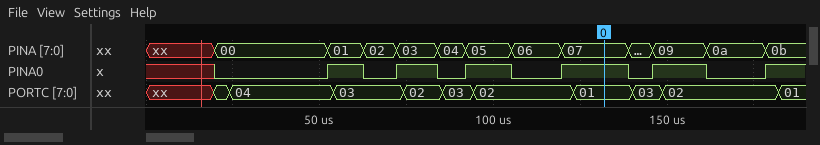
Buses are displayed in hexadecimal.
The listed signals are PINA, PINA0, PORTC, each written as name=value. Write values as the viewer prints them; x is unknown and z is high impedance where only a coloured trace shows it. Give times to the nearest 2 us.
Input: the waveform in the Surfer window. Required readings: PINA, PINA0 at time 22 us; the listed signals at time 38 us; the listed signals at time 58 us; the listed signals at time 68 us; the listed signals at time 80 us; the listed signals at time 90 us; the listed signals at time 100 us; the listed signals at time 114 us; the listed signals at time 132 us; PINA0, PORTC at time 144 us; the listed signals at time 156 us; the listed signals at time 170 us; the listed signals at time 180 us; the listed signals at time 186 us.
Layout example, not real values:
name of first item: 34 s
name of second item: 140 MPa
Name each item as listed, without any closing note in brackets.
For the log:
PINA, PINA0 at time 22 us: PINA=00, PINA0=0
the listed signals at time 38 us: PINA=00, PINA0=0, PORTC=04
the listed signals at time 58 us: PINA=01, PINA0=1, PORTC=03
the listed signals at time 68 us: PINA=02, PINA0=0, PORTC=03
the listed signals at time 80 us: PINA=03, PINA0=1, PORTC=02
the listed signals at time 90 us: PINA=04, PINA0=0, PORTC=03
the listed signals at time 100 us: PINA=05, PINA0=1, PORTC=02
the listed signals at time 114 us: PINA=06, PINA0=0, PORTC=02
the listed signals at time 132 us: PINA=07, PINA0=1, PORTC=01
PINA0, PORTC at time 144 us: PINA0=0, PORTC=03
the listed signals at time 156 us: PINA=09, PINA0=1, PORTC=02
the listed signals at time 170 us: PINA=0a, PINA0=0, PORTC=02
the listed signals at time 180 us: PINA=0b, PINA0=1, PORTC=02
the listed signals at time 186 us: PINA=0b, PINA0=1, PORTC=01
